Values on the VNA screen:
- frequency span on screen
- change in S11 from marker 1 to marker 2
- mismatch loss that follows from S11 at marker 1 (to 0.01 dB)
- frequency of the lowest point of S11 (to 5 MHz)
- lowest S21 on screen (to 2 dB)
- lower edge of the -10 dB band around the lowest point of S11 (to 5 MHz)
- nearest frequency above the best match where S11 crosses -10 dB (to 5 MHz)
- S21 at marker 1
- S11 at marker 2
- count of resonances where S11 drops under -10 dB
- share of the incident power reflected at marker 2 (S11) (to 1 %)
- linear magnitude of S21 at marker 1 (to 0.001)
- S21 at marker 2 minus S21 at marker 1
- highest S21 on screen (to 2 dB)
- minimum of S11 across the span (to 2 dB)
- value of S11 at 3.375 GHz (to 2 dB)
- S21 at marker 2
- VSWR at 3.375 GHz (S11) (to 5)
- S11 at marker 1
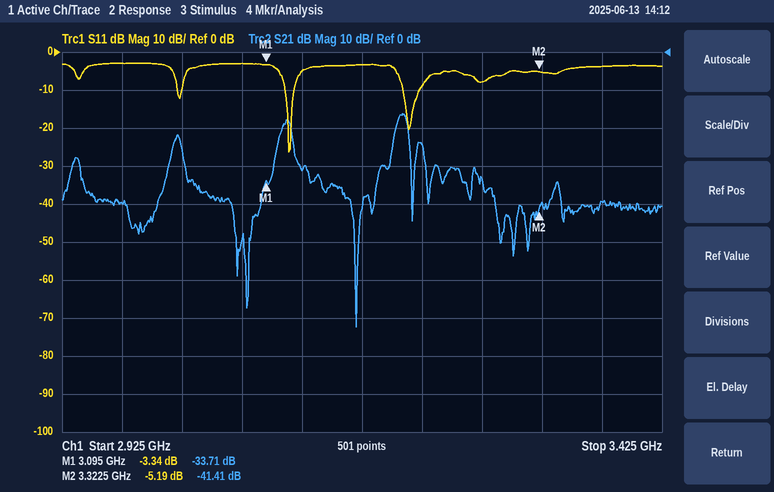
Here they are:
500 MHz
-1.85 dB
2.70 dB
3.115 GHz
-72 dB
3.110 GHz
3.120 GHz
-33.71 dB
-5.19 dB
3
30 %
0.021
-7.70 dB
-16 dB
-26 dB
-4 dB
-41.41 dB
5
-3.34 dB
